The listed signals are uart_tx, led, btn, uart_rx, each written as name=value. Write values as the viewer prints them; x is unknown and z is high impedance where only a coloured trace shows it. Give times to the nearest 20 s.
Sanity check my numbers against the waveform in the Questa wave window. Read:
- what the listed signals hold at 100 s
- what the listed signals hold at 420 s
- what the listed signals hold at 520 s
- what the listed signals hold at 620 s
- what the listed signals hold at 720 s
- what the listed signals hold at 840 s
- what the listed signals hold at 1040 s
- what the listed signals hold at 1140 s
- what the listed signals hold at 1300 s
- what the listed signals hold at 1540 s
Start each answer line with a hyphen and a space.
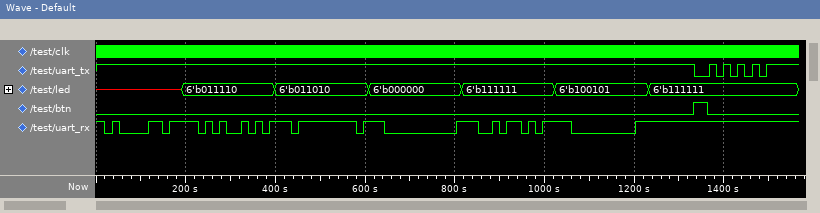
- uart_tx=1, led=x, btn=0, uart_rx=0
- uart_tx=1, led=6'b011010, btn=0, uart_rx=1
- uart_tx=1, led=6'b011010, btn=0, uart_rx=1
- uart_tx=1, led=6'b000000, btn=0, uart_rx=1
- uart_tx=1, led=6'b000000, btn=0, uart_rx=0
- uart_tx=1, led=6'b111111, btn=0, uart_rx=1
- uart_tx=1, led=6'b100101, btn=0, uart_rx=1
- uart_tx=1, led=6'b100101, btn=0, uart_rx=0
- uart_tx=1, led=6'b111111, btn=0, uart_rx=1
- uart_tx=1, led=6'b111111, btn=0, uart_rx=1
